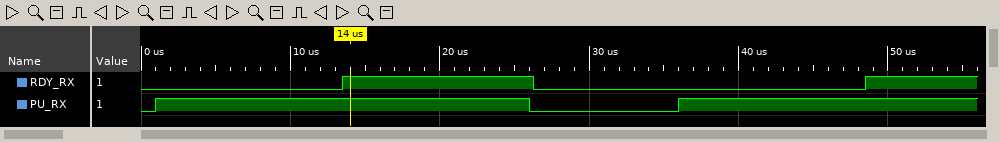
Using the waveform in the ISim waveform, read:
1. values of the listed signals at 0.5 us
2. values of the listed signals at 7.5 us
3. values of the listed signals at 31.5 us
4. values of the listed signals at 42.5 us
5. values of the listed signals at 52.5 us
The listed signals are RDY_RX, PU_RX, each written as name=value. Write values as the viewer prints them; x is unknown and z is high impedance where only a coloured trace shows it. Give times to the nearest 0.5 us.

RDY_RX=0, PU_RX=0
RDY_RX=0, PU_RX=1
RDY_RX=0, PU_RX=0
RDY_RX=0, PU_RX=1
RDY_RX=1, PU_RX=1
